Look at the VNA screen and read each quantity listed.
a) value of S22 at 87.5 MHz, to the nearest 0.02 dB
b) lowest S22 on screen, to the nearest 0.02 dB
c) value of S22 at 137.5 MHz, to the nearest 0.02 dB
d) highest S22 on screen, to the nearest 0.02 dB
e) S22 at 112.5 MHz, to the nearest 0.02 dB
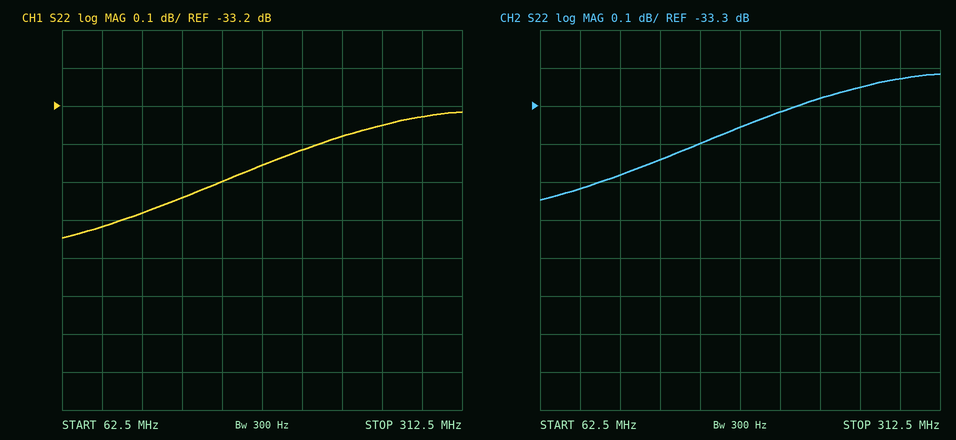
-33.52 dB
-33.54 dB
-33.44 dB
-33.22 dB
-33.48 dB
